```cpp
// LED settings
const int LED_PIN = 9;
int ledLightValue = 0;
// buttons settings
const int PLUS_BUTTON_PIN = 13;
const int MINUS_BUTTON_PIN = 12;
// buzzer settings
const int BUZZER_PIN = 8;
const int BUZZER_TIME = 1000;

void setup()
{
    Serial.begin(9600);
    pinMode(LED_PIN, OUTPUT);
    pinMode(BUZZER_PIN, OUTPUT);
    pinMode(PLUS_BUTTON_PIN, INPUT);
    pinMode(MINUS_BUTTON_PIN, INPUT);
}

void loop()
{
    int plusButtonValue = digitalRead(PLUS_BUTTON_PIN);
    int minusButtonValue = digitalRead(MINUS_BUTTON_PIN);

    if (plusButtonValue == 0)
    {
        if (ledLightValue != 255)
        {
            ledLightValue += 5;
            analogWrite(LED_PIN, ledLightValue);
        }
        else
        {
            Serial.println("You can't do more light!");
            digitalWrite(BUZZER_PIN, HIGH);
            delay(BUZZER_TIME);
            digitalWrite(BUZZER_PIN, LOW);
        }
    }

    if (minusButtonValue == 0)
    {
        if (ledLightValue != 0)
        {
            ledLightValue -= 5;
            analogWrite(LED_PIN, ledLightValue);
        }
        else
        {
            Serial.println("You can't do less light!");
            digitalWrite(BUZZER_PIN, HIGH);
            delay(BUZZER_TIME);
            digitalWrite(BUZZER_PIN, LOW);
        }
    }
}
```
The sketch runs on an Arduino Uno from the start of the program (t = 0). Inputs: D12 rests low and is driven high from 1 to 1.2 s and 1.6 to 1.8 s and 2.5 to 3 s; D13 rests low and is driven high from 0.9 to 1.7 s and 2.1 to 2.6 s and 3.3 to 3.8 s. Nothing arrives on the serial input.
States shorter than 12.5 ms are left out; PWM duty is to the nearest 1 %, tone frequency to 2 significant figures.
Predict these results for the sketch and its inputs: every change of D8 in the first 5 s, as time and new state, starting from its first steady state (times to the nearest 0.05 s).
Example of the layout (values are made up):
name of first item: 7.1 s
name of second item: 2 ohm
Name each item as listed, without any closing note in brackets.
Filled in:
every change of D8 in the first 5 s, as time and new state, starting from its first steady state: 0 s low; 0.9 s high; 1.9 s low; 2.1 s high; 3.1 s low; 3.3 s high; 4.3 s low
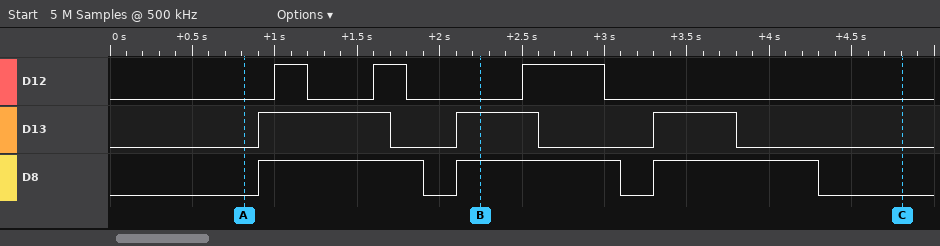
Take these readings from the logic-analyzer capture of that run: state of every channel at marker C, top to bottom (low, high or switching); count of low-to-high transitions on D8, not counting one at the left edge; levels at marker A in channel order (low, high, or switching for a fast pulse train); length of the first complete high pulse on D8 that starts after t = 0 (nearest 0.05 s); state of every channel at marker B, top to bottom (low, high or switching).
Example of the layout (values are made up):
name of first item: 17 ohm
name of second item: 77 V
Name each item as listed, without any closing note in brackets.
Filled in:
state of every channel at marker C, top to bottom: D12 low, D13 low, D8 low
count of low-to-high transitions on D8, not counting one at the left edge: 3
levels at marker A in channel order: D12 low, D13 low, D8 low
length of the first complete high pulse on D8 that starts after t = 0: 1.00 s
state of every channel at marker B, top to bottom: D12 low, D13 high, D8 high
